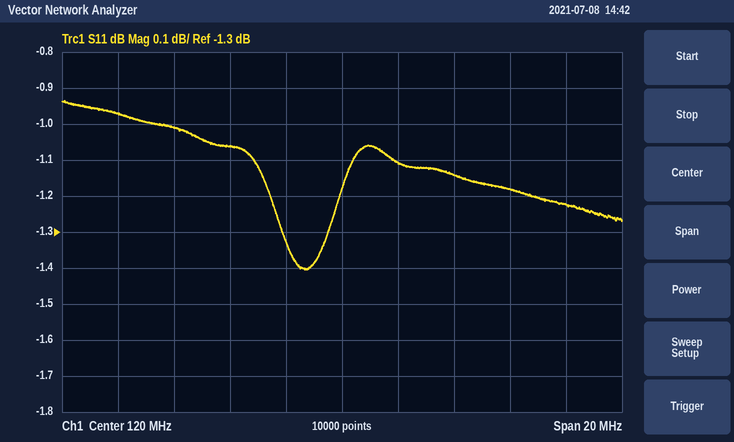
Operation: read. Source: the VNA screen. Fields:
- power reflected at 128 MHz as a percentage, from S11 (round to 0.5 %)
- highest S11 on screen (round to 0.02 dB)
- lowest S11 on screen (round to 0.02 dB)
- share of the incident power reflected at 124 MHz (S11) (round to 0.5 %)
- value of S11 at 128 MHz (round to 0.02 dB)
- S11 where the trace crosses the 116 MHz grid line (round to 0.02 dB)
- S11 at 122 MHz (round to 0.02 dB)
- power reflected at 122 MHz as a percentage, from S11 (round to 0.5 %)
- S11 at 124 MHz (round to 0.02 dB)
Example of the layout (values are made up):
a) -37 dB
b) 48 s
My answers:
a) 75.5 %
b) -0.94 dB
c) -1.40 dB
d) 77.0 %
e) -1.22 dB
f) -1.06 dB
g) -1.10 dB
h) 77.5 %
i) -1.14 dB
